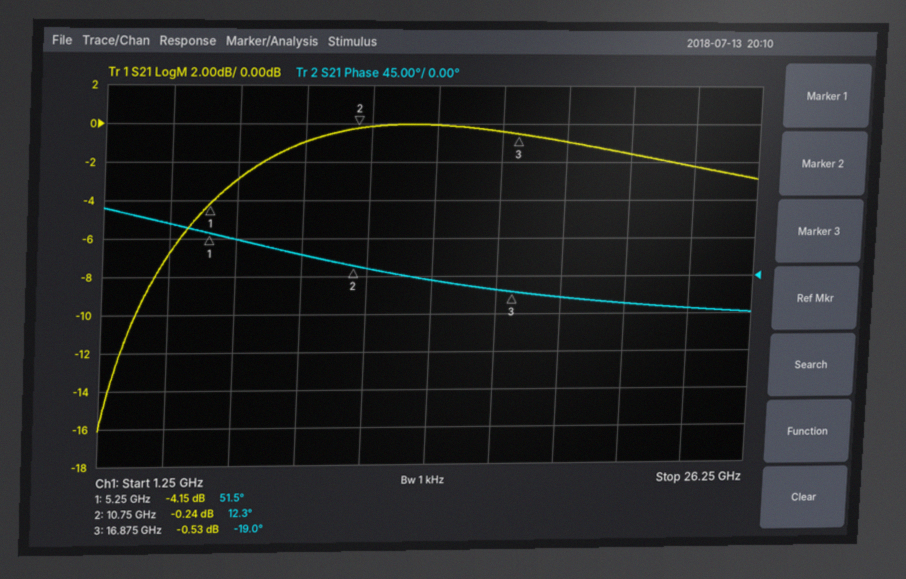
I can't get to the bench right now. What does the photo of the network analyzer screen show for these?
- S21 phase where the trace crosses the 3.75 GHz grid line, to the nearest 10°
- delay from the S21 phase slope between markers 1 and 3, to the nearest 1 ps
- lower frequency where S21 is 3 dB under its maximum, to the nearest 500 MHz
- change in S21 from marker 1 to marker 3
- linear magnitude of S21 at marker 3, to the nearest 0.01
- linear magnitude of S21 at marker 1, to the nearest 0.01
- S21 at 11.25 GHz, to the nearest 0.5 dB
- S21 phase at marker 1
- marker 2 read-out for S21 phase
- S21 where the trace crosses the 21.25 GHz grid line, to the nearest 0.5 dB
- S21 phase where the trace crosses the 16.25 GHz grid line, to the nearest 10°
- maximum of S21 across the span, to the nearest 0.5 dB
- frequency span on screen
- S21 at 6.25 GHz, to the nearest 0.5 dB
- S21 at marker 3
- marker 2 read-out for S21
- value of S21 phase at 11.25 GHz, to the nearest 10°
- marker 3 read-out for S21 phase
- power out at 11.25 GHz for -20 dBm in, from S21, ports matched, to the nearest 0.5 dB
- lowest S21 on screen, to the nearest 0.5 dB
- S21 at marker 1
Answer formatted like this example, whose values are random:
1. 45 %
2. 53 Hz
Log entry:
1. 60°
2. 17 ps
3. 6.0 GHz
4. 3.62 dB
5. 0.94
6. 0.62
7. 0.0 dB
8. 51.5°
9. 12.3°
10. -1.5 dB
11. -20°
12. 0.0 dB
13. 25 GHz
14. -3.0 dB
15. -0.53 dB
16. -0.24 dB
17. 10°
18. -19.0°
19. -20.0 dBm
20. -16.0 dB
21. -4.15 dB
